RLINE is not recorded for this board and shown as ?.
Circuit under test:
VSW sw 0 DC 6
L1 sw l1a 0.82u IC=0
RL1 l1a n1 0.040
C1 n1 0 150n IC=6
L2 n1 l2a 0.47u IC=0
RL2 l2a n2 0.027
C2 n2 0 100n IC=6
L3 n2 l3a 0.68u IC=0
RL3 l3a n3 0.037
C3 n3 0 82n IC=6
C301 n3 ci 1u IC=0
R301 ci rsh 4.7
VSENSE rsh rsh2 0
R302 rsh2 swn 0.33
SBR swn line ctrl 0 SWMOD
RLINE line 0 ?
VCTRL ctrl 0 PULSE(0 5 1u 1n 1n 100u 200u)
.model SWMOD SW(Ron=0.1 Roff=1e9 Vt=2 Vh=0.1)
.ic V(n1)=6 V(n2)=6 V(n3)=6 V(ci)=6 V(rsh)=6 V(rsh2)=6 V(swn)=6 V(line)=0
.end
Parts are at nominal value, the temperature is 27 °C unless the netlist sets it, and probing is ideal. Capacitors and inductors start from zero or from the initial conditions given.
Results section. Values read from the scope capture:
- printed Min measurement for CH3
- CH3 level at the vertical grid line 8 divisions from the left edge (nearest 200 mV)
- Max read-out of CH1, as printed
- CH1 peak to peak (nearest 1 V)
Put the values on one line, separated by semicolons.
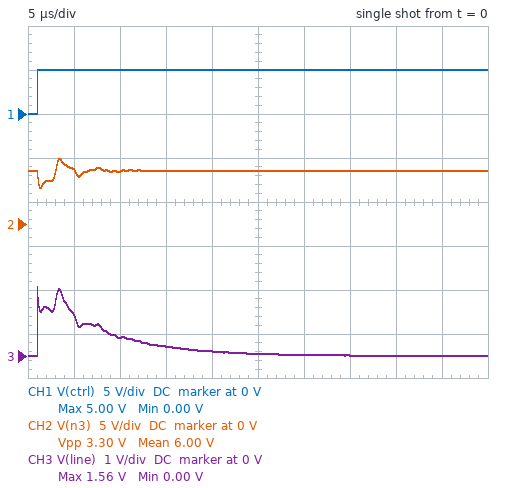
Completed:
0.00 V; 0 V; 5.00 V; 5 V
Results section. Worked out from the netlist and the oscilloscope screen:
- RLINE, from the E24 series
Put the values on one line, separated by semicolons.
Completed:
1.8 Ω
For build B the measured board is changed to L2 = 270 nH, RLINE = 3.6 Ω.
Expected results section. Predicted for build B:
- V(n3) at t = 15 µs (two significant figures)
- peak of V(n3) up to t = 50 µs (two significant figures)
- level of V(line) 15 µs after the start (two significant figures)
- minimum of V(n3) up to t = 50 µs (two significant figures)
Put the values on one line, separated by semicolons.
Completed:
6.0 V; 7.1 V; 510 mV; 4.4 V
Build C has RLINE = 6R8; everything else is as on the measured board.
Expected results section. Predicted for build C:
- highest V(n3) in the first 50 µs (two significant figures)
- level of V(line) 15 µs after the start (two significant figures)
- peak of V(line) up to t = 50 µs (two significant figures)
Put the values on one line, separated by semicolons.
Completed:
7.1 V; 1.1 V; 3.5 V
